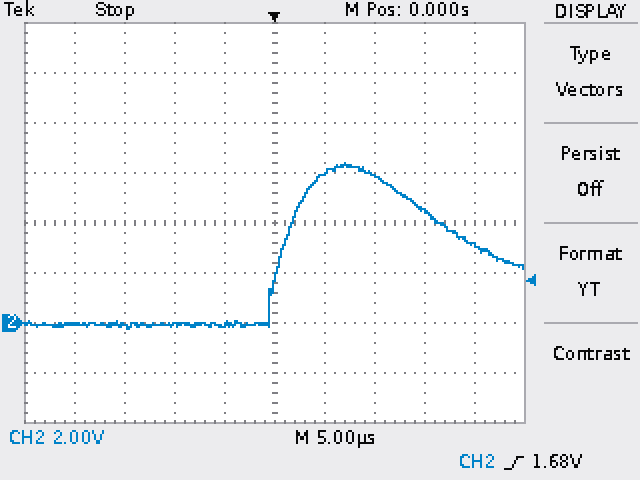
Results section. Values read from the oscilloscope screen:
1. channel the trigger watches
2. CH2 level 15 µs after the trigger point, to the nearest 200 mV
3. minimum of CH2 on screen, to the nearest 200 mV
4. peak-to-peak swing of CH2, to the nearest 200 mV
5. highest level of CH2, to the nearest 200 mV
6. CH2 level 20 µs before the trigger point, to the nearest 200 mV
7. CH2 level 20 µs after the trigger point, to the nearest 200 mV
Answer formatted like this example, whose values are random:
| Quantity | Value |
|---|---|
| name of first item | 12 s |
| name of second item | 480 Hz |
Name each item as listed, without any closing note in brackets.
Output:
| Quantity | Value |
|---|---|
| channel the trigger watches | CH2 |
| CH2 level 15 µs after the trigger point, to the nearest 200 mV | 4.6 V |
| minimum of CH2 on screen, to the nearest 200 mV | -200 mV |
| peak-to-peak swing of CH2, to the nearest 200 mV | 6.6 V |
| highest level of CH2, to the nearest 200 mV | 6.4 V |
| CH2 level 20 µs before the trigger point, to the nearest 200 mV | 0.0 V |
| CH2 level 20 µs after the trigger point, to the nearest 200 mV | 3.2 V |
